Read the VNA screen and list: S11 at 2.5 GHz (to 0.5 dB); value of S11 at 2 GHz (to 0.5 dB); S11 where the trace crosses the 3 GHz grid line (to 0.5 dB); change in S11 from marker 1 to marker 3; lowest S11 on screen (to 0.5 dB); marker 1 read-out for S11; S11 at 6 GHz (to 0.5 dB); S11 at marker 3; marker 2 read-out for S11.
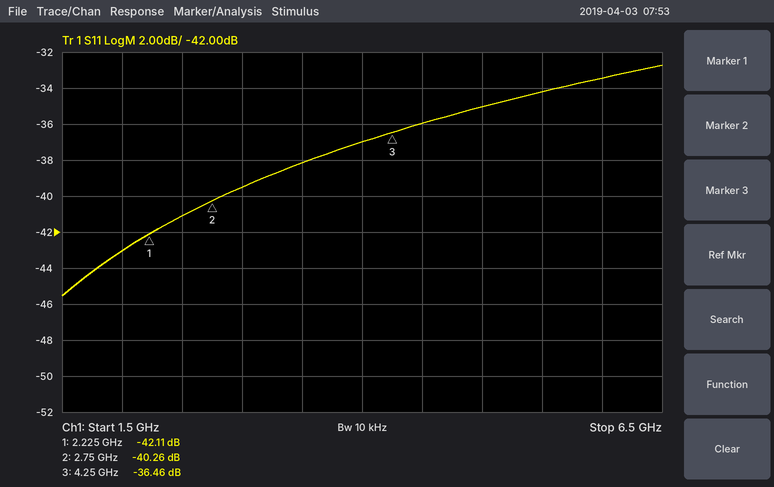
-41.0 dB
-43.0 dB
-39.5 dB
5.65 dB
-45.5 dB
-42.11 dB
-33.5 dB
-36.46 dB
-40.26 dB
